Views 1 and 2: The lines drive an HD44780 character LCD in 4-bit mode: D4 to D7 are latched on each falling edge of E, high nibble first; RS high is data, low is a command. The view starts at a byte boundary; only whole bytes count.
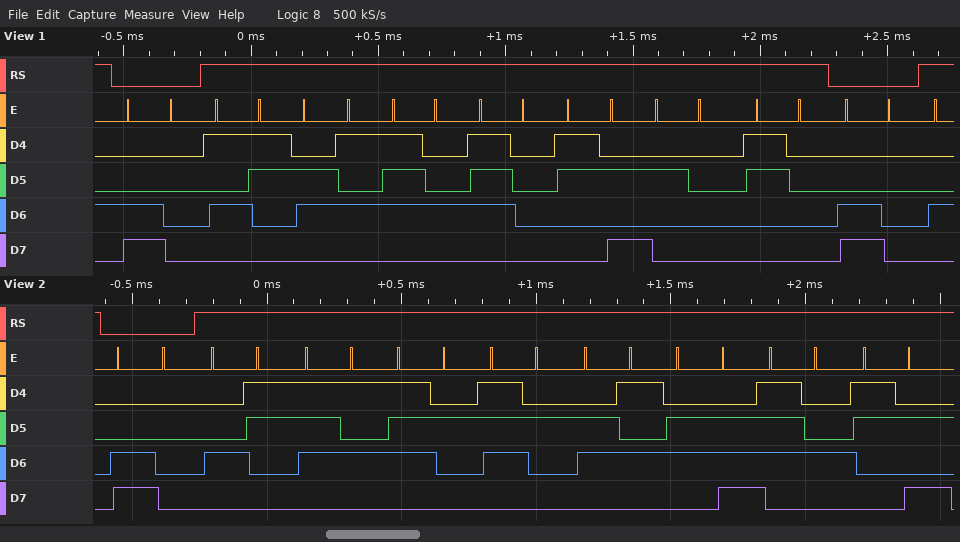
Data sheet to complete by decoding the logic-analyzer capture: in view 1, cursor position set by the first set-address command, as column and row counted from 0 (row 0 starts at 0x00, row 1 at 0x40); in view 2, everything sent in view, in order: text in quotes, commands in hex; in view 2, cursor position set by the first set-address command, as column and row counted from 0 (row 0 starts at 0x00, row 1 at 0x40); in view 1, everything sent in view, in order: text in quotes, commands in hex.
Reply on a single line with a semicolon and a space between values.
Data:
column 0, row 1; 0xC0 "Current:"; column 0, row 1; 0xC0 "Setp: 0" 0xC0
